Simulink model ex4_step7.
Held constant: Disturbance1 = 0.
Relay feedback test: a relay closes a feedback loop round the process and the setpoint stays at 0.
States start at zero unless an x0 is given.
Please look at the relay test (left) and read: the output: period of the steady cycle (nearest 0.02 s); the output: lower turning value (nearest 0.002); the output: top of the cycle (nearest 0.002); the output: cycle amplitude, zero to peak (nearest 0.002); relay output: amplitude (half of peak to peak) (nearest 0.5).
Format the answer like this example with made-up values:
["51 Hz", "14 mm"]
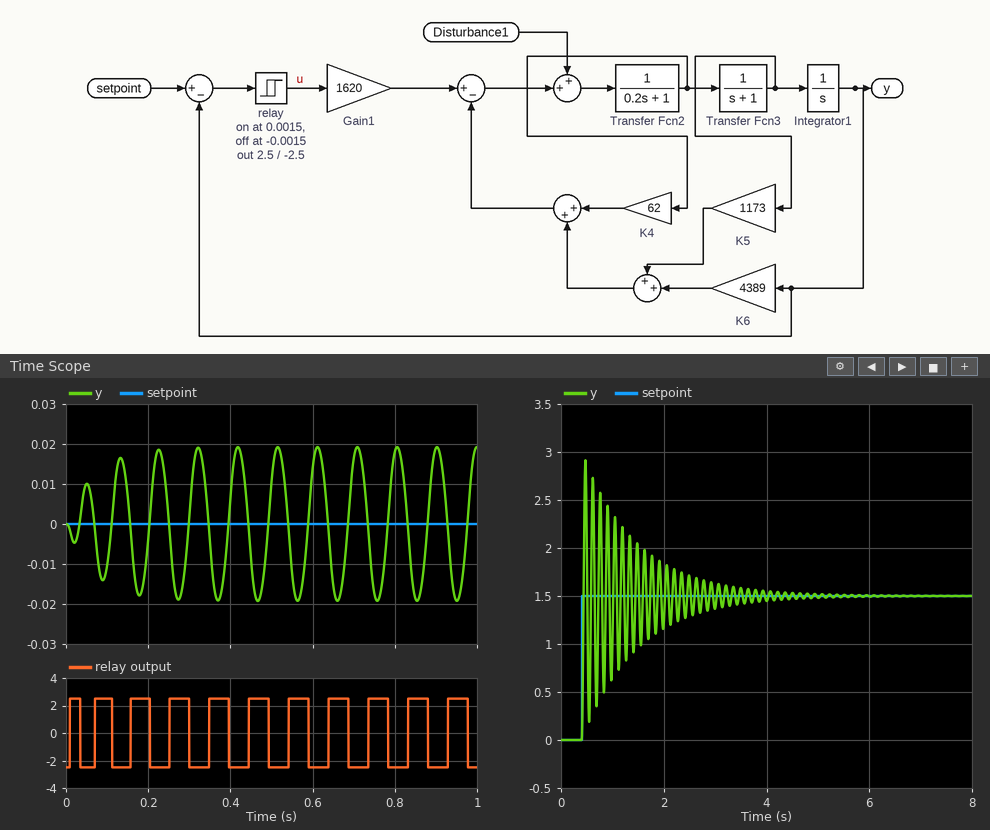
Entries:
["0.10 s", "-0.020", "0.020", "0.020", "2.5"]
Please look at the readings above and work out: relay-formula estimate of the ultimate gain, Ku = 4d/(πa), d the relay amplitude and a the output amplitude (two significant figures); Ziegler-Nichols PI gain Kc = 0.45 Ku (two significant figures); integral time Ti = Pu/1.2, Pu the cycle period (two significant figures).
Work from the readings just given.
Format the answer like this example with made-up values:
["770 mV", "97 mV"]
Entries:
["160", "72", "0.083 s"]
